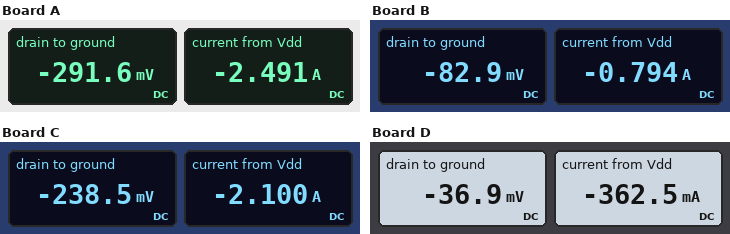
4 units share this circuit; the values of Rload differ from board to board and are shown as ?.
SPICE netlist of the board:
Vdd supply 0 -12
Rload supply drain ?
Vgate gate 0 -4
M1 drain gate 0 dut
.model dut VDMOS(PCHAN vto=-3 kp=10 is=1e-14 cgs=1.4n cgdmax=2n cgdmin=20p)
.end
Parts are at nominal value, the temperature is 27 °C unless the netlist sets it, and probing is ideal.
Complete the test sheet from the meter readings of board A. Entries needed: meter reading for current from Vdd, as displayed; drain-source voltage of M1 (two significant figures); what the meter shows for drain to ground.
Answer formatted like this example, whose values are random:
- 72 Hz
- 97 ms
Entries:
- -2.491 A
- -290 mV
- -291.6 mV
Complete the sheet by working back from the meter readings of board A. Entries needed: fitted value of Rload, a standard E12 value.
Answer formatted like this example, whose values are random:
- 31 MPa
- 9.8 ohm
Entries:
- 4.7 Ω
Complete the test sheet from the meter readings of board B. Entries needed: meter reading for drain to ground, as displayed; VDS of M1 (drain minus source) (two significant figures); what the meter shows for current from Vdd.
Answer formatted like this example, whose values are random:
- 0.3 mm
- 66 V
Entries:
- -82.9 mV
- -83 mV
- -0.794 A
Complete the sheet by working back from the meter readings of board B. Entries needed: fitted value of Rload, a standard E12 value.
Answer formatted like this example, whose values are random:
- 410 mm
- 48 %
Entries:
- 15 Ω
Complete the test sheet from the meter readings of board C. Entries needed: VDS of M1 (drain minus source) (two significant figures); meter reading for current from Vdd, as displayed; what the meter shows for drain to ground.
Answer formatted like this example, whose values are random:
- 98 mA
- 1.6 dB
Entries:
- -240 mV
- -2.100 A
- -238.5 mV
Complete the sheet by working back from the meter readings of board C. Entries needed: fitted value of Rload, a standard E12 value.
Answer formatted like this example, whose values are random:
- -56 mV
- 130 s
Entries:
- 5.6 Ω
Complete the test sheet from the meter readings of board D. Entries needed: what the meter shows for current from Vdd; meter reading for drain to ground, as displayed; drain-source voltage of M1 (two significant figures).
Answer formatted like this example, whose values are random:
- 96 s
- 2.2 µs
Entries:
- -362.5 mA
- -36.9 mV
- -37 mV
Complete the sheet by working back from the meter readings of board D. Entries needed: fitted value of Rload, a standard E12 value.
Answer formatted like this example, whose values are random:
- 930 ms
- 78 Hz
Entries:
- 33 Ω
